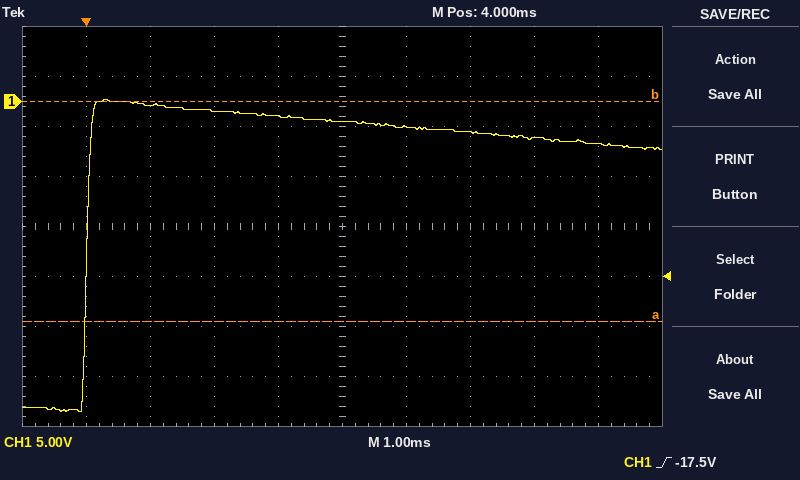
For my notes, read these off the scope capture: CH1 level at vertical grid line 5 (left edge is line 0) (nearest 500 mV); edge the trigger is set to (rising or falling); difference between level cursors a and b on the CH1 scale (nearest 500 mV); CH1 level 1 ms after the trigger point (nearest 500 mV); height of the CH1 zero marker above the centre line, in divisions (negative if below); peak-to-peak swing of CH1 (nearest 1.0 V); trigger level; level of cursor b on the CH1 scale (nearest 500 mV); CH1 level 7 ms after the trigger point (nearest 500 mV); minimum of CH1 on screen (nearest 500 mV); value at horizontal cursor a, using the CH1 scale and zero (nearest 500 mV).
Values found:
-2.0 V
rising
22.0 V
-500 mV
+2.5 div
31.0 V
-17.5 V
0.0 V
-3.5 V
-31.0 V
-22.0 V
